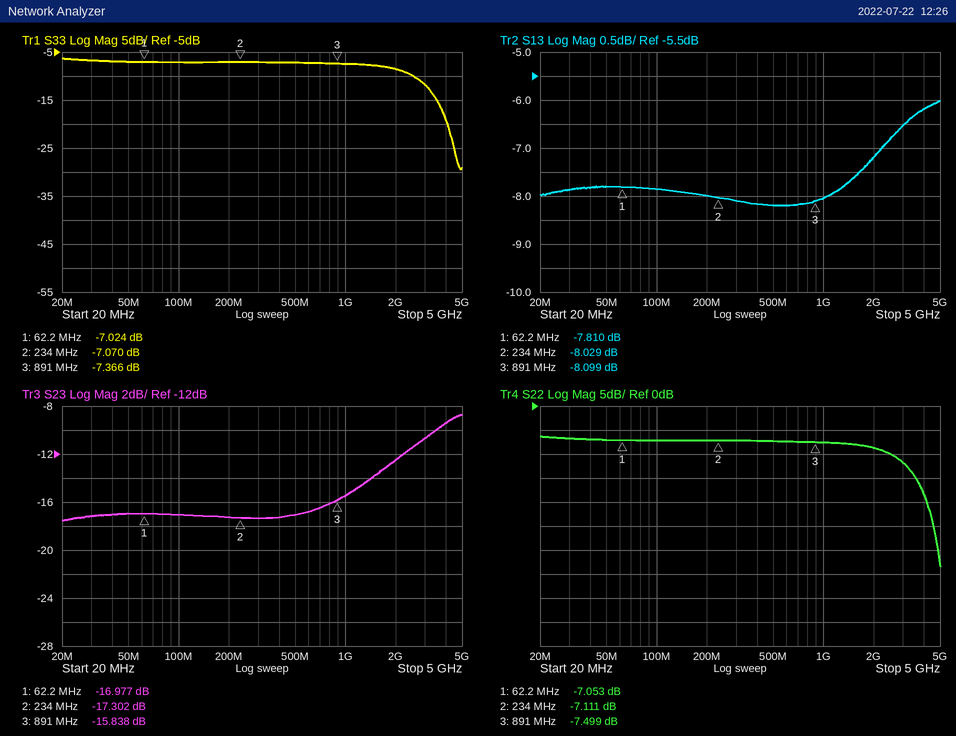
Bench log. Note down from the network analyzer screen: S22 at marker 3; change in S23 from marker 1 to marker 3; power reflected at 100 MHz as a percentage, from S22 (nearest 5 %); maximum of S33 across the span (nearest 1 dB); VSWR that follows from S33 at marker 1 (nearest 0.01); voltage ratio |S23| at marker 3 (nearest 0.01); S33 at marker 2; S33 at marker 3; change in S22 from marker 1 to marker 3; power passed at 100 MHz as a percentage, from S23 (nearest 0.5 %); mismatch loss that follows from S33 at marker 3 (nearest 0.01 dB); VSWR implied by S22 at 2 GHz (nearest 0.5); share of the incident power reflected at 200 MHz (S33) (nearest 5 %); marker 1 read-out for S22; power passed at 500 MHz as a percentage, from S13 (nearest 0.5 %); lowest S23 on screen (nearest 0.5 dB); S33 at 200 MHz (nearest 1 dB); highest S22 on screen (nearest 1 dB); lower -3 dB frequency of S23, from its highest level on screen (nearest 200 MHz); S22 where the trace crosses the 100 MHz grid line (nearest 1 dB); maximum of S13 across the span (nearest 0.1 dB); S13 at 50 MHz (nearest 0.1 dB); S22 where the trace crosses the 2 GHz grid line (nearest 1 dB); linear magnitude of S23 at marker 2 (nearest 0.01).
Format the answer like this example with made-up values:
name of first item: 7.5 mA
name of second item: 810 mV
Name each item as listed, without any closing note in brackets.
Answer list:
S22 at marker 3: -7.499 dB
change in S23 from marker 1 to marker 3: 1.139 dB
power reflected at 100 MHz as a percentage, from S22: 20 %
maximum of S33 across the span: -6 dB
VSWR that follows from S33 at marker 1: 2.61
voltage ratio |S23| at marker 3: 0.16
S33 at marker 2: -7.070 dB
S33 at marker 3: -7.366 dB
change in S22 from marker 1 to marker 3: -0.446 dB
power passed at 100 MHz as a percentage, from S23: 2.0 %
mismatch loss that follows from S33 at marker 3: 0.88 dB
VSWR implied by S22 at 2 GHz: 2.0
share of the incident power reflected at 200 MHz (S33): 20 %
marker 1 read-out for S22: -7.053 dB
power passed at 500 MHz as a percentage, from S13: 15.0 %
lowest S23 on screen: -17.5 dB
S33 at 200 MHz: -7 dB
highest S22 on screen: -6 dB
lower -3 dB frequency of S23, from its highest level on screen: 2.4 GHz
S22 where the trace crosses the 100 MHz grid line: -7 dB
maximum of S13 across the span: -6.0 dB
S13 at 50 MHz: -7.8 dB
S22 where the trace crosses the 2 GHz grid line: -9 dB
linear magnitude of S23 at marker 2: 0.14
